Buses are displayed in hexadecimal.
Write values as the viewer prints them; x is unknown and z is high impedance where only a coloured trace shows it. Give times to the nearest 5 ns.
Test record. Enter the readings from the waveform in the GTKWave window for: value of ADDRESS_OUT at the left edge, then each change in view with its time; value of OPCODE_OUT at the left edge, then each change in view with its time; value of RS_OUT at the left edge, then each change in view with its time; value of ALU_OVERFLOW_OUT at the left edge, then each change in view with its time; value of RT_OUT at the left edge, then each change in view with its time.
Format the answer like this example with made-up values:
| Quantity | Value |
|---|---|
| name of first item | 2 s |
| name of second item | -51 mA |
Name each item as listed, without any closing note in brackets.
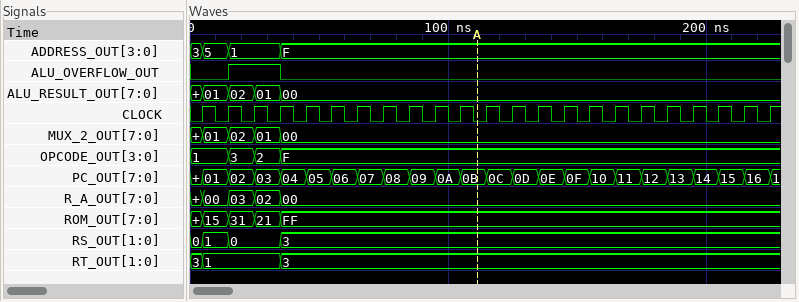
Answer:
| Quantity | Value |
|---|---|
| value of ADDRESS_OUT at the left edge, then each change in view with its time | 3, 5 at 5 ns, 1 at 15 ns, F at 35 ns |
| value of OPCODE_OUT at the left edge, then each change in view with its time | 1, 3 at 15 ns, 2 at 25 ns, F at 35 ns |
| value of RS_OUT at the left edge, then each change in view with its time | 0, 1 at 5 ns, 0 at 15 ns, 3 at 35 ns |
| value of ALU_OVERFLOW_OUT at the left edge, then each change in view with its time | 0, 1 at 15 ns, 0 at 35 ns |
| value of RT_OUT at the left edge, then each change in view with its time | 3, 1 at 5 ns, 3 at 35 ns |
